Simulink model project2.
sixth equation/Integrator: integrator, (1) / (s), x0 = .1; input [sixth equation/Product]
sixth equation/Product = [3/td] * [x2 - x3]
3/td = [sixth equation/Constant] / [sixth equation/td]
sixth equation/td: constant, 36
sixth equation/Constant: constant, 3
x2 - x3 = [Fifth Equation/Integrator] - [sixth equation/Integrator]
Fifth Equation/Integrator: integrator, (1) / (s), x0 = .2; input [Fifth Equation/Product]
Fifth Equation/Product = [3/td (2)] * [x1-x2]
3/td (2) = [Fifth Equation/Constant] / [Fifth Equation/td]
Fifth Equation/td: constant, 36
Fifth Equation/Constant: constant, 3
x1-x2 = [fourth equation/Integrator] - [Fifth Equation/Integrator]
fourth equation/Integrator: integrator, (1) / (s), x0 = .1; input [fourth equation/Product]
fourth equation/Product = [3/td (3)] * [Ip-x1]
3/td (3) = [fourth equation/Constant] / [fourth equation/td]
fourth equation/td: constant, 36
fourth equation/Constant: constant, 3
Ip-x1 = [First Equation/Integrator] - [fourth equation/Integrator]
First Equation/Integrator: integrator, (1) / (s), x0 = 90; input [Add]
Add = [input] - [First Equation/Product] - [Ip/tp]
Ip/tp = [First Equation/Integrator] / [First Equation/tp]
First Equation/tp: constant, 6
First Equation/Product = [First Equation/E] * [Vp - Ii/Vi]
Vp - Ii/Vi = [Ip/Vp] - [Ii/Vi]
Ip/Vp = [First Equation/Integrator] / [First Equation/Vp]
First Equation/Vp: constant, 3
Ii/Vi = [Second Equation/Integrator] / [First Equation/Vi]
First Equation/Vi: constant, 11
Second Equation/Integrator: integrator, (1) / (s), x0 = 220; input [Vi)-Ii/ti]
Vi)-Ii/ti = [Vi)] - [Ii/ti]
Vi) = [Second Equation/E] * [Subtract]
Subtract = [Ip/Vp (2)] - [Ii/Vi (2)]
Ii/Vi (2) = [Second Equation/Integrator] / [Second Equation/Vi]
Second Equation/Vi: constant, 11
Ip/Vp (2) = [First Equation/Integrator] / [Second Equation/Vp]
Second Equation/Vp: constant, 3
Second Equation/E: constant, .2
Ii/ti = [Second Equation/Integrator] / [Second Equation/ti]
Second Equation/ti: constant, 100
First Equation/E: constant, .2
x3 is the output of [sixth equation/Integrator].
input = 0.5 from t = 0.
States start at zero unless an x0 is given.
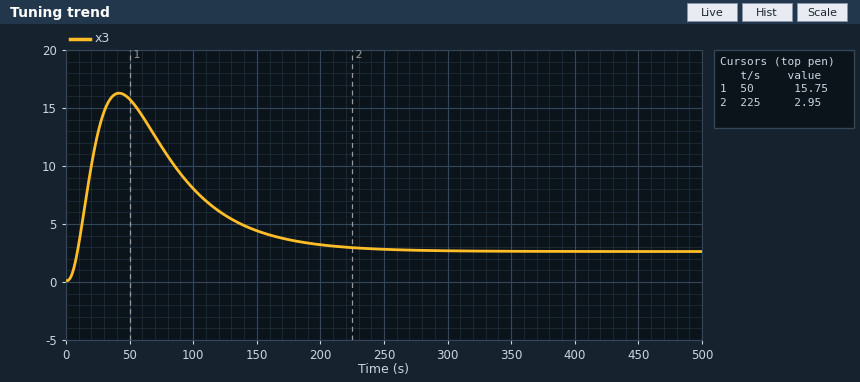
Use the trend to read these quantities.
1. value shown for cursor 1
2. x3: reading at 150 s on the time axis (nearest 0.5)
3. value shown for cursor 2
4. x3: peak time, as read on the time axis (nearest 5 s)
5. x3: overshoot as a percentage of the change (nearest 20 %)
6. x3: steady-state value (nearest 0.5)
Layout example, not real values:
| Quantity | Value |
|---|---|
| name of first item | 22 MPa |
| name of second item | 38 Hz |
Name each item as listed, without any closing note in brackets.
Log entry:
| Quantity | Value |
|---|---|
| value shown for cursor 1 | 15.75 |
| x3: reading at 150 s on the time axis | 4.5 |
| value shown for cursor 2 | 2.95 |
| x3: peak time, as read on the time axis | 40 s |
| x3: overshoot as a percentage of the change | 540 % |
| x3: steady-state value | 2.5 |
